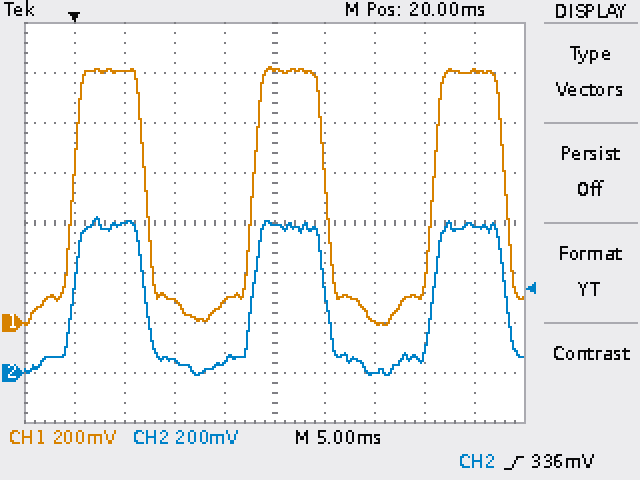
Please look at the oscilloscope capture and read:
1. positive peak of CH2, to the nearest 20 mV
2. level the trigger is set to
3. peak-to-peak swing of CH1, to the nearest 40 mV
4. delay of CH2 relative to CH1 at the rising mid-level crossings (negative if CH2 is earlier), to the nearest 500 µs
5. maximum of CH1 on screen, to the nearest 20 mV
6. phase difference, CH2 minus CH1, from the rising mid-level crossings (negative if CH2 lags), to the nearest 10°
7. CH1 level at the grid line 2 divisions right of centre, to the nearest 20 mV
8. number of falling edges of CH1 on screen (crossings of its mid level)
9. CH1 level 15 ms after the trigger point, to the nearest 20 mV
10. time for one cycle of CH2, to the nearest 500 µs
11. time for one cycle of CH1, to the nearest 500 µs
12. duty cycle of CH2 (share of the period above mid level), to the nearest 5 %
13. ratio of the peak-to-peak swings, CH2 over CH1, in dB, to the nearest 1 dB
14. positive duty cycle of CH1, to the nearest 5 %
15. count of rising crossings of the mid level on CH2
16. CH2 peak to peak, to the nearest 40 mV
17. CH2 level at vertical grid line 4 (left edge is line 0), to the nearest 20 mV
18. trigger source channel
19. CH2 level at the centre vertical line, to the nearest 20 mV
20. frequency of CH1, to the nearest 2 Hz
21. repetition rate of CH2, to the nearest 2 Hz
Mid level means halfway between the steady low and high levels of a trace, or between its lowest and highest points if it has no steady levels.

620 mV
336 mV
1.04 V
0.0 ms
1.02 V
0°
0 mV
3
80 mV
18.0 ms
18.0 ms
40 %
-4 dB
40 %
3
640 mV
40 mV
CH2
600 mV
56 Hz
56 Hz
